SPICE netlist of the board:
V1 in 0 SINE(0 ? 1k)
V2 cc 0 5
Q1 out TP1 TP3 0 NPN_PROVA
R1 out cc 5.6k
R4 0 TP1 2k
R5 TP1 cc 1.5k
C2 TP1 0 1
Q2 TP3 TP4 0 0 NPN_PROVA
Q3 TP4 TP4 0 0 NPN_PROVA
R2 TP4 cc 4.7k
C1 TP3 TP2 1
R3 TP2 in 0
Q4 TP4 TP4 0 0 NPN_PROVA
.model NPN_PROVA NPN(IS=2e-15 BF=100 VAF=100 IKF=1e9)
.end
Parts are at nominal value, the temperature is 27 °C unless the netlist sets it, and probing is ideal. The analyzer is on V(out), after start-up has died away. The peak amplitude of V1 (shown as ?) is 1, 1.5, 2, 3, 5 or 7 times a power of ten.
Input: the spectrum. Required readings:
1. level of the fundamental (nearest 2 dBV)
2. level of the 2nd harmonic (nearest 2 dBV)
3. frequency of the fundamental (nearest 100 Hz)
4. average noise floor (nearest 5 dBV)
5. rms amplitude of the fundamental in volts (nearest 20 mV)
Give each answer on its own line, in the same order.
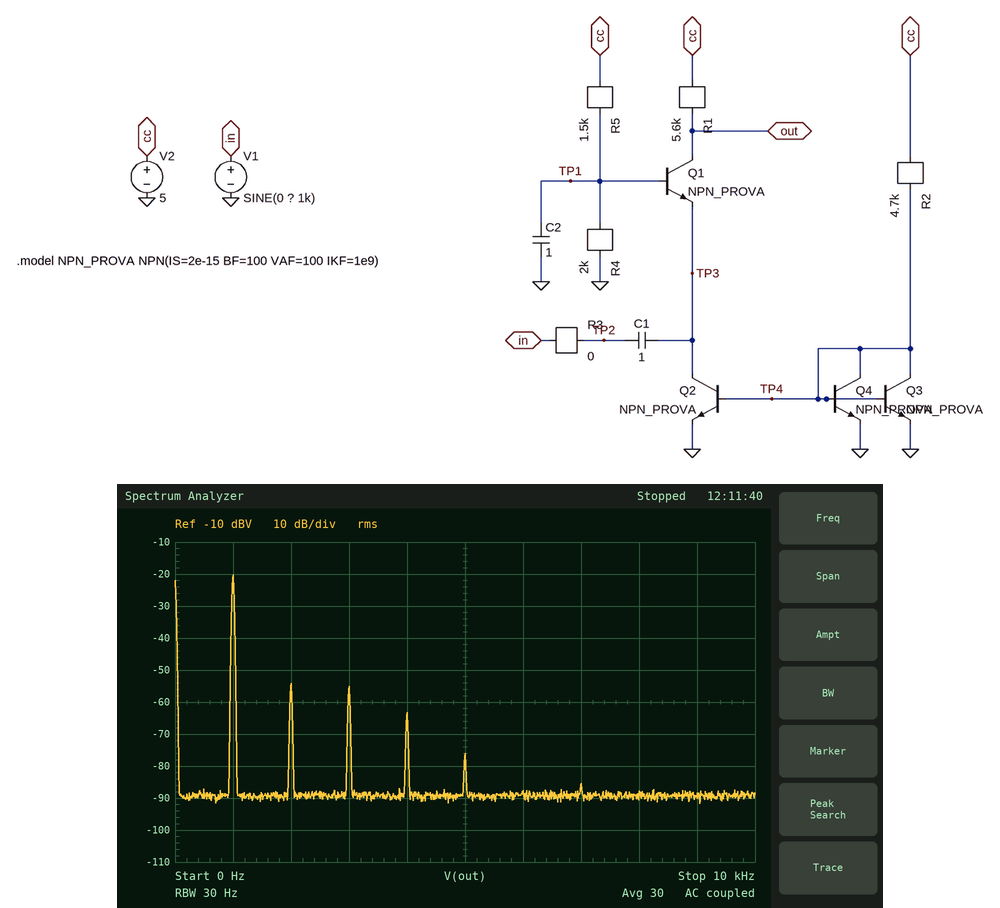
-20 dBV
-54 dBV
1.0 kHz
-90 dBV
100 mV
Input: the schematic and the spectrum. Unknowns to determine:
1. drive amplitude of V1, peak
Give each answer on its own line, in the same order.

1.5 mV
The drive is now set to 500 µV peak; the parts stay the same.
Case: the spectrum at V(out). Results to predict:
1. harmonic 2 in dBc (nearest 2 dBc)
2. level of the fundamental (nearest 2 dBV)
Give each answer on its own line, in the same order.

-56 dBc
-30 dBV
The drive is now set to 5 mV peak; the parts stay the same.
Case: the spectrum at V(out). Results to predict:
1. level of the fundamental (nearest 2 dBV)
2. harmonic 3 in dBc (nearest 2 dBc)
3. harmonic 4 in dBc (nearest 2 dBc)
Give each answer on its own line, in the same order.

-12 dBV
-22 dBc
-38 dBc
